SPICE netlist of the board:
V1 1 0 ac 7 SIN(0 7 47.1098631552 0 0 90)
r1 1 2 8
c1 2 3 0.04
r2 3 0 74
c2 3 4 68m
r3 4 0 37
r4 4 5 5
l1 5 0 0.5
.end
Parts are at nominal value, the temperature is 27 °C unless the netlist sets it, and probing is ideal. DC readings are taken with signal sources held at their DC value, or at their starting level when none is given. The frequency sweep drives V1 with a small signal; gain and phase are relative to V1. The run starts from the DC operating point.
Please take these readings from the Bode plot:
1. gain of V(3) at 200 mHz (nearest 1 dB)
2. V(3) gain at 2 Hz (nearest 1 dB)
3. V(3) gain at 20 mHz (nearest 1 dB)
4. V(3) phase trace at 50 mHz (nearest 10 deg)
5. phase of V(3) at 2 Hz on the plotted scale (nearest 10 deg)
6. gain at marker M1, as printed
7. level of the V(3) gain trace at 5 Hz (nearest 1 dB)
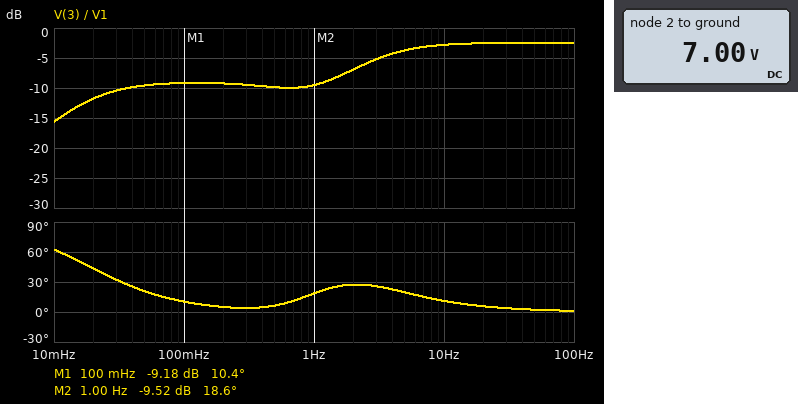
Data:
-9 dB
-7 dB
-12 dB
20 deg
30 deg
-9.18 dB
-4 dB
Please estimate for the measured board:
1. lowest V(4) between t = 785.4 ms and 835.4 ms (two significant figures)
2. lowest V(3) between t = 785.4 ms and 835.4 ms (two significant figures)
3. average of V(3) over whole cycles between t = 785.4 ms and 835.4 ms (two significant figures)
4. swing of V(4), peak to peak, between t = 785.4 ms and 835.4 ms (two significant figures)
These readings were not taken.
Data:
-5.3 V
-7.5 V
-2.2 V
11 V
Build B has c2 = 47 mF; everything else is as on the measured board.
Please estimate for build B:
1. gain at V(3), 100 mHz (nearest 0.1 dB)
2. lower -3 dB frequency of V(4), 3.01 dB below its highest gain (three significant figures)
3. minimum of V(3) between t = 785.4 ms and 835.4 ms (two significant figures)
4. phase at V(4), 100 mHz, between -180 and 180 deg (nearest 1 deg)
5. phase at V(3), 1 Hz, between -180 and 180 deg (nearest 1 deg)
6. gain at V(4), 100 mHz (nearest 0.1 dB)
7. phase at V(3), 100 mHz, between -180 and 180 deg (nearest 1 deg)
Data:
-7.4 dB
2.28 Hz
-8.0 V
97 deg
10 deg
-25.1 dB
11 deg
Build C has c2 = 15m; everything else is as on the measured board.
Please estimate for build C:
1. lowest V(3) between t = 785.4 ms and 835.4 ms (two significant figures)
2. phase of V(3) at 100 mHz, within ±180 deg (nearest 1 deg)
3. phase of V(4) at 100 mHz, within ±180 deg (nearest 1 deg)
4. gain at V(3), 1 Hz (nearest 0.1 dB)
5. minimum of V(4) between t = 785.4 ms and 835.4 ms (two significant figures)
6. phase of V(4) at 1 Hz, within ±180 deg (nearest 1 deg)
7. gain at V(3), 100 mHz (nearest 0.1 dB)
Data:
-9.3 V
18 deg
109 deg
-5.8 dB
-5.2 V
74 deg
-3.9 dB
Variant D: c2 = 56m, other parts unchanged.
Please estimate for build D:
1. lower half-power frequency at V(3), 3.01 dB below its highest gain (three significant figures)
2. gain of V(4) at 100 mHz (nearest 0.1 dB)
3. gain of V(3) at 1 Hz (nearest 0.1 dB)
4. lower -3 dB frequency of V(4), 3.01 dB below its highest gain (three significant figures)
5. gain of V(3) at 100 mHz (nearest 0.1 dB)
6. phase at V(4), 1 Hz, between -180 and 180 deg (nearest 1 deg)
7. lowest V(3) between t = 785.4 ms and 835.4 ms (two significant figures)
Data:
2.90 Hz
-24.4 dB
-9.6 dB
2.30 Hz
-8.2 dB
48 deg
-7.8 V
